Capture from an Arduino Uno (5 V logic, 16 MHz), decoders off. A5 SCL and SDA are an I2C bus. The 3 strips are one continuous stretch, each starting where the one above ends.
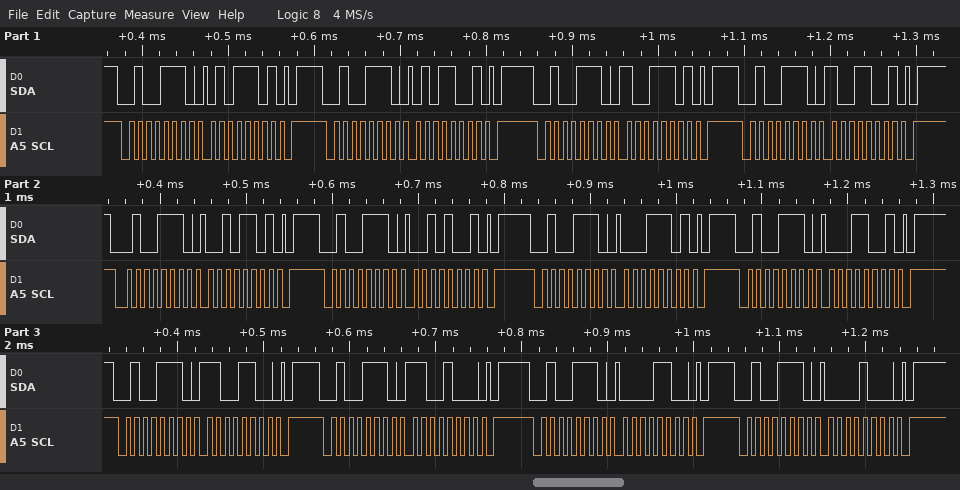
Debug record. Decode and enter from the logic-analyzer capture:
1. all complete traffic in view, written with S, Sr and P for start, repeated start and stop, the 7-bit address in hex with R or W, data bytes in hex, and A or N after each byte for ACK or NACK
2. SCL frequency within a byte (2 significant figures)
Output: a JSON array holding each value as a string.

["S 27W A 5D A P S 27W A 59 A P S 27W A 9D A P S 27W A 99 A P S 27W A 2D A P S 27W A 29 A P S 27W A 1D A P S 27W A 19 A P S 27W A CC A P S 27W A C8 A P S 27W A 0C A P S 27W A 08 A P", "100 kHz"]
